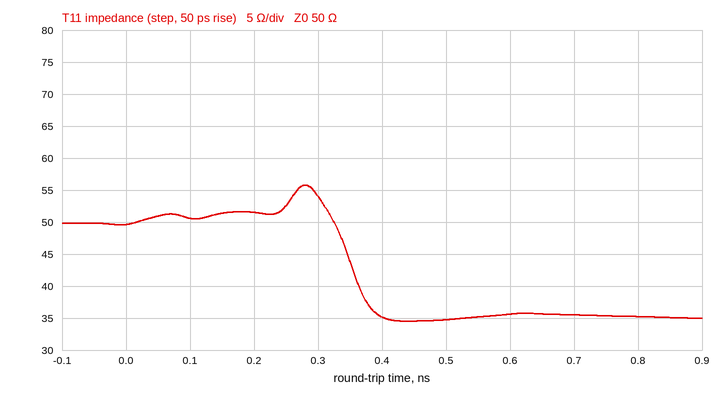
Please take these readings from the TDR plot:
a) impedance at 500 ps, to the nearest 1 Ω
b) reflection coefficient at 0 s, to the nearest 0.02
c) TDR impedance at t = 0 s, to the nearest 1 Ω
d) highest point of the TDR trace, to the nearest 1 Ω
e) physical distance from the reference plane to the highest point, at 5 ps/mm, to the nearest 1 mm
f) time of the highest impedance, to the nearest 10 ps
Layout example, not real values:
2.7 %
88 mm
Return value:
35 Ω
0.00
50 Ω
56 Ω
28 mm
280 ps
